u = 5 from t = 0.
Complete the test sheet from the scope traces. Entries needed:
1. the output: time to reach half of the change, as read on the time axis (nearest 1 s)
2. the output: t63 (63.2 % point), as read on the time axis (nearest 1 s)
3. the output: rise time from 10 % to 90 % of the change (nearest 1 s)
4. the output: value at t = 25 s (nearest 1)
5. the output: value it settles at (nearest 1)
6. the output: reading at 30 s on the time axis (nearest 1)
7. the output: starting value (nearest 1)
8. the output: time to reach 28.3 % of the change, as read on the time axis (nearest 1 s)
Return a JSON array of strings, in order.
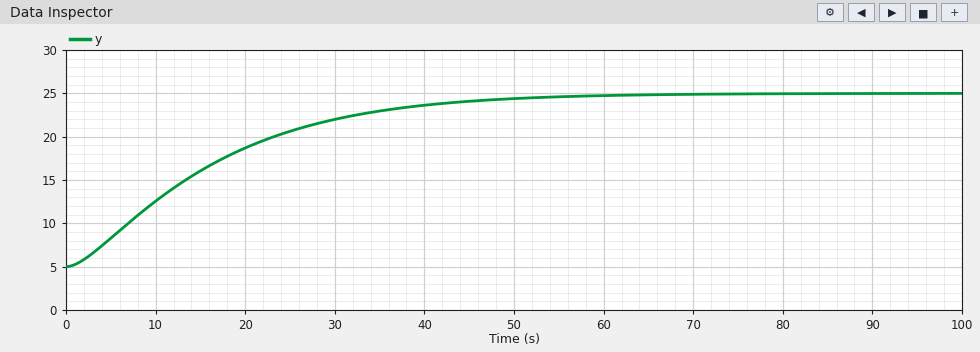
["13 s", "18 s", "32 s", "21", "25", "22", "5", "8 s"]
